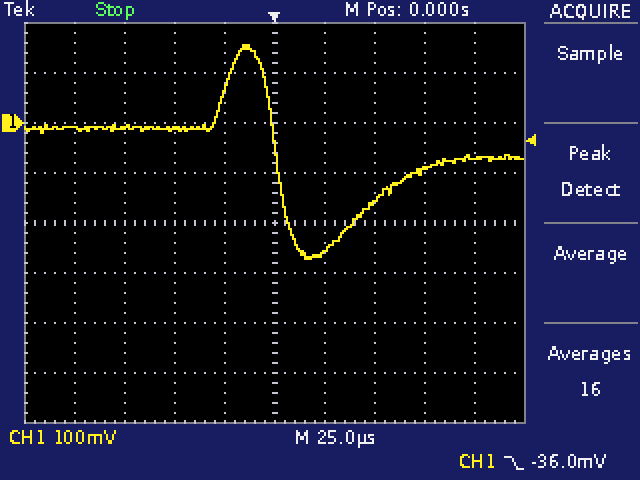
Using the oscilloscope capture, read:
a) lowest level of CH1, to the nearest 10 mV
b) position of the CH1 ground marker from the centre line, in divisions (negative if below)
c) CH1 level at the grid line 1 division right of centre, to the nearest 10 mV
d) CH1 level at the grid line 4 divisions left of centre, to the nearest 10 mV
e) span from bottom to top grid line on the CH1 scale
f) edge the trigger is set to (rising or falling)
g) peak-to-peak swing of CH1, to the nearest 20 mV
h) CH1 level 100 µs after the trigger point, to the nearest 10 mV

-270 mV
+2.0 div
-260 mV
-10 mV
800 mV
falling
420 mV
-70 mV
